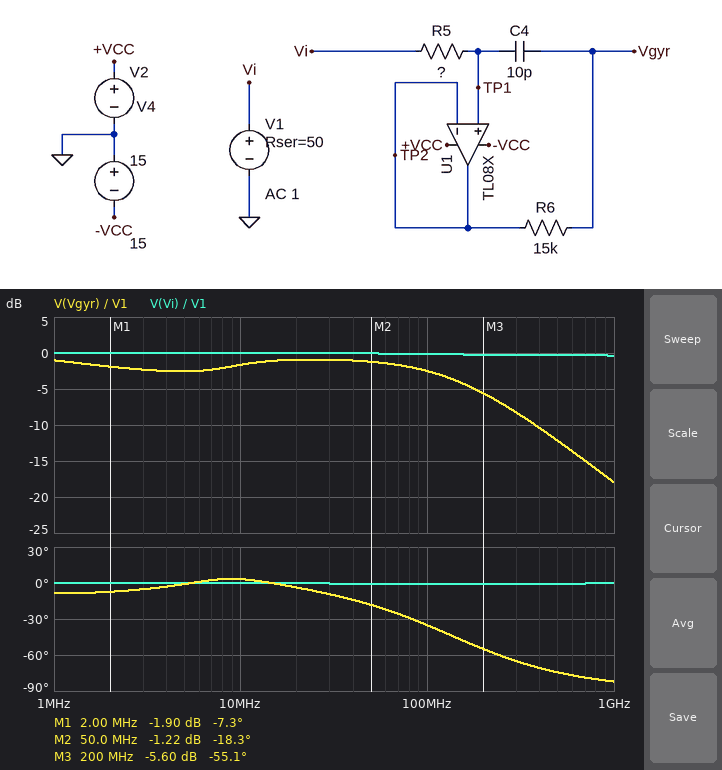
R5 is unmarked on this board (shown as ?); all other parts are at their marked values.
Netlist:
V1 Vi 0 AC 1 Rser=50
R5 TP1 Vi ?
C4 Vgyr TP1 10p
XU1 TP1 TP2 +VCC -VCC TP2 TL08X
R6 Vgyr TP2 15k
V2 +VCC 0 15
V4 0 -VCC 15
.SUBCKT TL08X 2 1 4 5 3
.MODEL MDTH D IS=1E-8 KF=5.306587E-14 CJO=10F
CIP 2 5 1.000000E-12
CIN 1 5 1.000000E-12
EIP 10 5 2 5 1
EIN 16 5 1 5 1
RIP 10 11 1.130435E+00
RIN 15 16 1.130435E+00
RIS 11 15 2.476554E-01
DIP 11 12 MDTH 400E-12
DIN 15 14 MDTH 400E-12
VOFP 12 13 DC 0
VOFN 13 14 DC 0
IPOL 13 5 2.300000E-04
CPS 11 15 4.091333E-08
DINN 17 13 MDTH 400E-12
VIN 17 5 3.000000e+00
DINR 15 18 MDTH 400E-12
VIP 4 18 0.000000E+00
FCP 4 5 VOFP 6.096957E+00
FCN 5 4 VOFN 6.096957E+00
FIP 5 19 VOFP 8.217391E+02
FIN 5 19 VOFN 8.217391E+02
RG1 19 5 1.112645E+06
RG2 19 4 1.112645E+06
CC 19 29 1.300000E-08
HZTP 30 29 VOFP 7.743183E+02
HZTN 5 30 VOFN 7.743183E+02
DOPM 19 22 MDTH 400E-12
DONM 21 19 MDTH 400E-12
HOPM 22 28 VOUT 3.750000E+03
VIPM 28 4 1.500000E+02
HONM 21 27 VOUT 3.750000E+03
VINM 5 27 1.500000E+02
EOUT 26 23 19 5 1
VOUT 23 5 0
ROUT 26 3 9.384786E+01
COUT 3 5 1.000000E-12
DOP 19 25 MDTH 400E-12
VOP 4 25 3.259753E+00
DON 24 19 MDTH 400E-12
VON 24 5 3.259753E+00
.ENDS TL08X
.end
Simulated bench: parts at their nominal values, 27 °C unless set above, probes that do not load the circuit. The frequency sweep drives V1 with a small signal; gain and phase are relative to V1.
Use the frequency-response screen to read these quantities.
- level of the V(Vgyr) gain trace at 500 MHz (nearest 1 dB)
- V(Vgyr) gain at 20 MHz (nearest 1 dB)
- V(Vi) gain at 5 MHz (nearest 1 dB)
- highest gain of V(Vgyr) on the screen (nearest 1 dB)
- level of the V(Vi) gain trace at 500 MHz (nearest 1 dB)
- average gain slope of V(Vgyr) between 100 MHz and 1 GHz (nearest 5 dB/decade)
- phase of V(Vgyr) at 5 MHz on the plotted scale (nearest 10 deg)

-12 dB
-1 dB
0 dB
-1 dB
0 dB
-15 dB/decade
0 deg
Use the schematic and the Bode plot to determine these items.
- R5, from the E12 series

1.2 kΩ
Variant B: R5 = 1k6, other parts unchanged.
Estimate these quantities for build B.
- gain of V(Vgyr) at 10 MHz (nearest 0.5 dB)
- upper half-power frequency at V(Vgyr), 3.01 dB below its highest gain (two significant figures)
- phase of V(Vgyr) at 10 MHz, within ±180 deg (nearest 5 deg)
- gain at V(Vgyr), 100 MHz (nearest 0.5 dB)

-2.0 dB
85 MHz
0 deg
-3.5 dB
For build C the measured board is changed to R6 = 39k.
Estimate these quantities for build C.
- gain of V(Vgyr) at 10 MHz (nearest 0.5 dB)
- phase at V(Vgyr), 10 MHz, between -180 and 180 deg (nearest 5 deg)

-0.5 dB
0 deg
